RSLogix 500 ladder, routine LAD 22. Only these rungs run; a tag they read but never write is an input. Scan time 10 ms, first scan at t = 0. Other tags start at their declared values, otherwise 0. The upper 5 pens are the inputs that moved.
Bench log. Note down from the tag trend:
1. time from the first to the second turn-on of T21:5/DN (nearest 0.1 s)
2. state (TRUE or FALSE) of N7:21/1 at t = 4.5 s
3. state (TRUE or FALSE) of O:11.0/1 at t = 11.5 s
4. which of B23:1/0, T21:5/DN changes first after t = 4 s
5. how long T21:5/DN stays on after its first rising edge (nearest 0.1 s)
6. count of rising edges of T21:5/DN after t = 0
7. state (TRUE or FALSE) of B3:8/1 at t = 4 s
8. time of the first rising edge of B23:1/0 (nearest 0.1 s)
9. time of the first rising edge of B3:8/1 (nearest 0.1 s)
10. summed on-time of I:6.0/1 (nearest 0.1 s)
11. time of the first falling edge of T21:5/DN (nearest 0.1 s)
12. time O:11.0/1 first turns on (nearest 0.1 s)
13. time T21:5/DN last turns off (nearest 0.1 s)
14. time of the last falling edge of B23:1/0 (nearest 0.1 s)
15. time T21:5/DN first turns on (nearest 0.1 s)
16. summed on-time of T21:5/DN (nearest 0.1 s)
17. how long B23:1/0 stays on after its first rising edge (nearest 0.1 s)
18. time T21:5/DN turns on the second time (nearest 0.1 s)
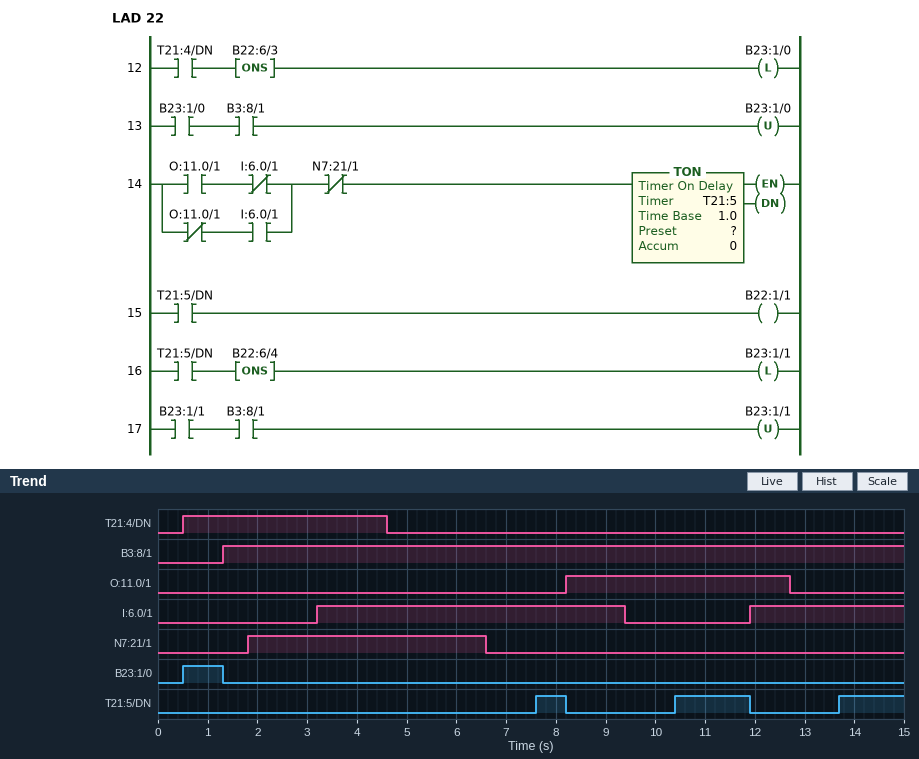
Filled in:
2.8 s
TRUE
TRUE
T21:5/DN
0.6 s
3
TRUE
0.5 s
1.3 s
9.3 s
8.2 s
8.2 s
11.9 s
1.3 s
7.6 s
3.4 s
0.8 s
10.4 s
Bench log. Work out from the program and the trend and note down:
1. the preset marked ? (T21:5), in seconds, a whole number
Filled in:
1 s
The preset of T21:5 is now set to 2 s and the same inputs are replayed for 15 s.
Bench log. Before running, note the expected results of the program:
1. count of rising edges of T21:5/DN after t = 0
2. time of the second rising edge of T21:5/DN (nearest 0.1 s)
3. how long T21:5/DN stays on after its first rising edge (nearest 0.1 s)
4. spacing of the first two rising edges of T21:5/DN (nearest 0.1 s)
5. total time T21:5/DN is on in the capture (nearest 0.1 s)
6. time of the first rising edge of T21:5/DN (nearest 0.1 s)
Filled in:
2
14.7 s
0.5 s
3.3 s
0.8 s
11.4 s
